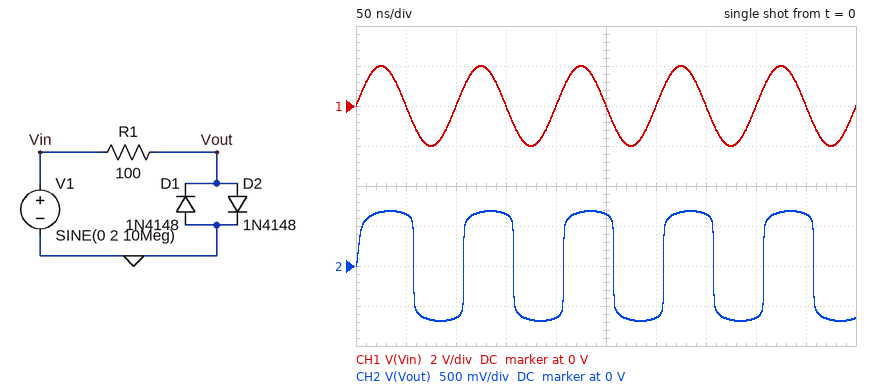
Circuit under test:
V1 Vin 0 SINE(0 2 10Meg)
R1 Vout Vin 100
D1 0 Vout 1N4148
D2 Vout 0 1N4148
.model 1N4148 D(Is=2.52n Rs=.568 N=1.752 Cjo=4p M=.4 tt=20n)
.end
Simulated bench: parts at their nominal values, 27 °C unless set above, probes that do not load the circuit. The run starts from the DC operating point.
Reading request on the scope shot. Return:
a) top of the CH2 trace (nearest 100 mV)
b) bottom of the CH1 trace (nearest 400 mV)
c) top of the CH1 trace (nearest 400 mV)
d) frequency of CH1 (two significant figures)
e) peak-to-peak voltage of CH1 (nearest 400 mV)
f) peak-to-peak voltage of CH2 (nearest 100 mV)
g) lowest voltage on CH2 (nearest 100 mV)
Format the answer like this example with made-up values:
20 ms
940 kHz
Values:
700 mV
-2.0 V
2.0 V
10 MHz
4.0 V
1.4 V
-700 mV
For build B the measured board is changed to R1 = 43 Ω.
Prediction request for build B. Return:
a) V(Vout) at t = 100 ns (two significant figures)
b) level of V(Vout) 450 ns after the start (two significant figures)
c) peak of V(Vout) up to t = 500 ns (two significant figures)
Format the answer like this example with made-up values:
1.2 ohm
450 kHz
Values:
-680 mV
680 mV
730 mV
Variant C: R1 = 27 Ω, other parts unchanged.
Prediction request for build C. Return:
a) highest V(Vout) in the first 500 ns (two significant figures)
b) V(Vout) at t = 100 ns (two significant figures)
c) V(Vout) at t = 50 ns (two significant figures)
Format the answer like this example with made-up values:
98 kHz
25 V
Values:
760 mV
-690 mV
690 mV
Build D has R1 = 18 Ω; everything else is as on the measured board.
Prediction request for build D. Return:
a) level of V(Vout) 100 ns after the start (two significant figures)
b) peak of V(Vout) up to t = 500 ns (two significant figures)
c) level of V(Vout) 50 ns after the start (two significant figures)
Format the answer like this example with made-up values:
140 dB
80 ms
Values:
-700 mV
790 mV
700 mV
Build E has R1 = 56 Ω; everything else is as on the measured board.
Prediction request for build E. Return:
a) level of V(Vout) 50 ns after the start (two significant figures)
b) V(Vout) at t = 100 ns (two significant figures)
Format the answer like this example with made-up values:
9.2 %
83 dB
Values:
670 mV
-670 mV
